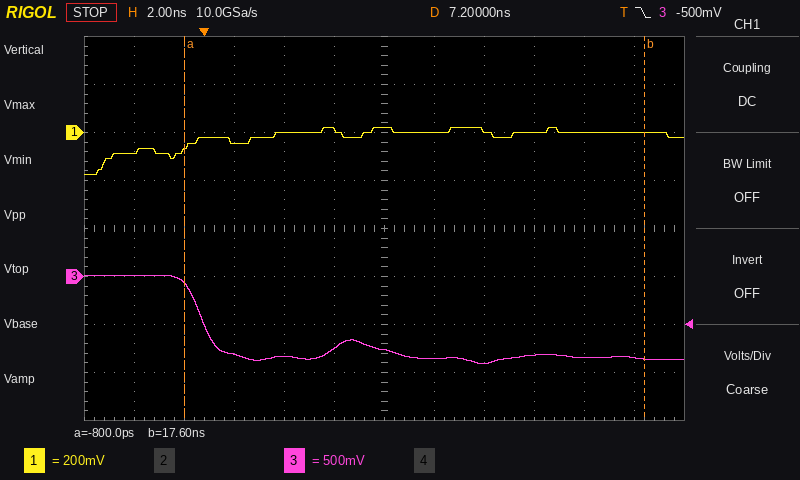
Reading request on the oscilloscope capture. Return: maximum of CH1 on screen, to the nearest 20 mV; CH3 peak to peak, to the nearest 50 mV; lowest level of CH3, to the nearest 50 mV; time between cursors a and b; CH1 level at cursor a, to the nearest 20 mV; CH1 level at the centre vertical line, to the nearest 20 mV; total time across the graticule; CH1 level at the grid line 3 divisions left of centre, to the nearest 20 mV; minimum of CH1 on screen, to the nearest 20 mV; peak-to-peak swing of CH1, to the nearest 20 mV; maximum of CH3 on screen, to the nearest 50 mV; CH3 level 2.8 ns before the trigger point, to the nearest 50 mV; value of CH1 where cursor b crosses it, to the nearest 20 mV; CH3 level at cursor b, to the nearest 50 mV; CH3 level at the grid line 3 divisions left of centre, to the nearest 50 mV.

20 mV
900 mV
-900 mV
18.4 ns
-60 mV
20 mV
24 ns
-40 mV
-180 mV
200 mV
0 mV
0 mV
0 mV
-850 mV
-800 mV
